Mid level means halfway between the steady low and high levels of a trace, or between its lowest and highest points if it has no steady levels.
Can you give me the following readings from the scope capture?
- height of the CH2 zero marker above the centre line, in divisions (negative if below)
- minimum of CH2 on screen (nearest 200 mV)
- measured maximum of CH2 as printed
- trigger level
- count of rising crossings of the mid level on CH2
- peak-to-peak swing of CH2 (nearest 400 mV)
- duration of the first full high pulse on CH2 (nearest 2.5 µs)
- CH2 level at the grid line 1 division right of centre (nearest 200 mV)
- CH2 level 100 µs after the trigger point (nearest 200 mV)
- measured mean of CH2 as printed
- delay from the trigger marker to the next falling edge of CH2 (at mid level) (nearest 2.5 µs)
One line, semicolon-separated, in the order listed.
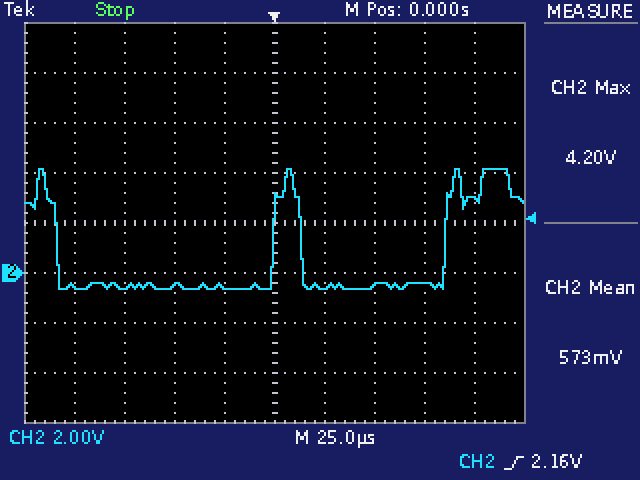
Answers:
-1.0 div; -600 mV; 4.20 V; 2.16 V; 2; 4.8 V; 12.5 µs; -600 mV; 3.0 V; 573 mV; 12.5 µs
